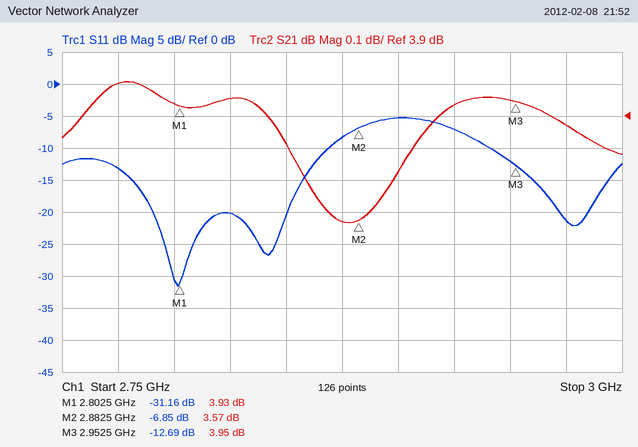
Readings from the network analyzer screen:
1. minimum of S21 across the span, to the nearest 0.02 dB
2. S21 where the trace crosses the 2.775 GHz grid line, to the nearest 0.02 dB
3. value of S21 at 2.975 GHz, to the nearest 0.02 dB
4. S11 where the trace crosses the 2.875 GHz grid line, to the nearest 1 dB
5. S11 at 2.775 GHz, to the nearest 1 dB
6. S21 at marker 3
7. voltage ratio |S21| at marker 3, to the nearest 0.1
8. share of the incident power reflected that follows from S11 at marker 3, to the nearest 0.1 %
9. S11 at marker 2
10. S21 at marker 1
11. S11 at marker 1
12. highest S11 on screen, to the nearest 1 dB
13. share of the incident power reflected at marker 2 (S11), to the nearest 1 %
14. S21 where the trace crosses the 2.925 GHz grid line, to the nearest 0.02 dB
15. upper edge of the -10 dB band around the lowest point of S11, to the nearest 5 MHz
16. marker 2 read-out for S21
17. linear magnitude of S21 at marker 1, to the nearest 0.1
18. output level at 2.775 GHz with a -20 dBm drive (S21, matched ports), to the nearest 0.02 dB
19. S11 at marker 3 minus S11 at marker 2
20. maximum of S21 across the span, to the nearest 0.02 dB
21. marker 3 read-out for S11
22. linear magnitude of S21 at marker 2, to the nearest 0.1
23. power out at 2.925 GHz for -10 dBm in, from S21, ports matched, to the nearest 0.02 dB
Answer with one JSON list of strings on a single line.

["3.56 dB", "4.00 dB", "3.88 dB", "-8 dB", "-13 dB", "3.95 dB", "1.6", "5.4 %", "-6.85 dB", "3.93 dB", "-31.16 dB", "-5 dB", "21 %", "3.94 dB", "2.870 GHz", "3.57 dB", "1.6", "-16.00 dBm", "-5.84 dB", "4.00 dB", "-12.69 dB", "1.5", "-6.06 dBm"]
